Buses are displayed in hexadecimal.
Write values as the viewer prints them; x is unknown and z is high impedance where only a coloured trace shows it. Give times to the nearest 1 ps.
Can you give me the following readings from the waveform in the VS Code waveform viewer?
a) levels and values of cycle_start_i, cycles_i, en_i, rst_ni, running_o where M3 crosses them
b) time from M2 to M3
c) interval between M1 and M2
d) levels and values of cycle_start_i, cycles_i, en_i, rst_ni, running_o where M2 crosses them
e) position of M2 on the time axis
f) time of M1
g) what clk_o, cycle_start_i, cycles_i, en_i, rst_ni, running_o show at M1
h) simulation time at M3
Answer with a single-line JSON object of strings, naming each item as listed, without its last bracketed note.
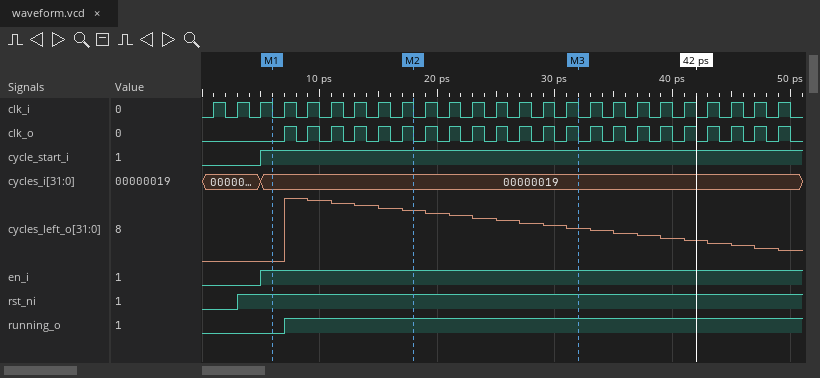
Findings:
{"levels and values of cycle_start_i, cycles_i, en_i, rst_ni, running_o where M3 crosses them": "cycle_start_i=1, cycles_i=00000019, en_i=1, rst_ni=1, running_o=1", "time from M2 to M3": "14 ps", "interval between M1 and M2": "12 ps", "levels and values of cycle_start_i, cycles_i, en_i, rst_ni, running_o where M2 crosses them": "cycle_start_i=1, cycles_i=00000019, en_i=1, rst_ni=1, running_o=1", "position of M2 on the time axis": "18 ps", "time of M1": "6 ps", "what clk_o, cycle_start_i, cycles_i, en_i, rst_ni, running_o show at M1": "clk_o=0, cycle_start_i=1, cycles_i=00000019, en_i=1, rst_ni=1, running_o=0", "simulation time at M3": "32 ps"}
